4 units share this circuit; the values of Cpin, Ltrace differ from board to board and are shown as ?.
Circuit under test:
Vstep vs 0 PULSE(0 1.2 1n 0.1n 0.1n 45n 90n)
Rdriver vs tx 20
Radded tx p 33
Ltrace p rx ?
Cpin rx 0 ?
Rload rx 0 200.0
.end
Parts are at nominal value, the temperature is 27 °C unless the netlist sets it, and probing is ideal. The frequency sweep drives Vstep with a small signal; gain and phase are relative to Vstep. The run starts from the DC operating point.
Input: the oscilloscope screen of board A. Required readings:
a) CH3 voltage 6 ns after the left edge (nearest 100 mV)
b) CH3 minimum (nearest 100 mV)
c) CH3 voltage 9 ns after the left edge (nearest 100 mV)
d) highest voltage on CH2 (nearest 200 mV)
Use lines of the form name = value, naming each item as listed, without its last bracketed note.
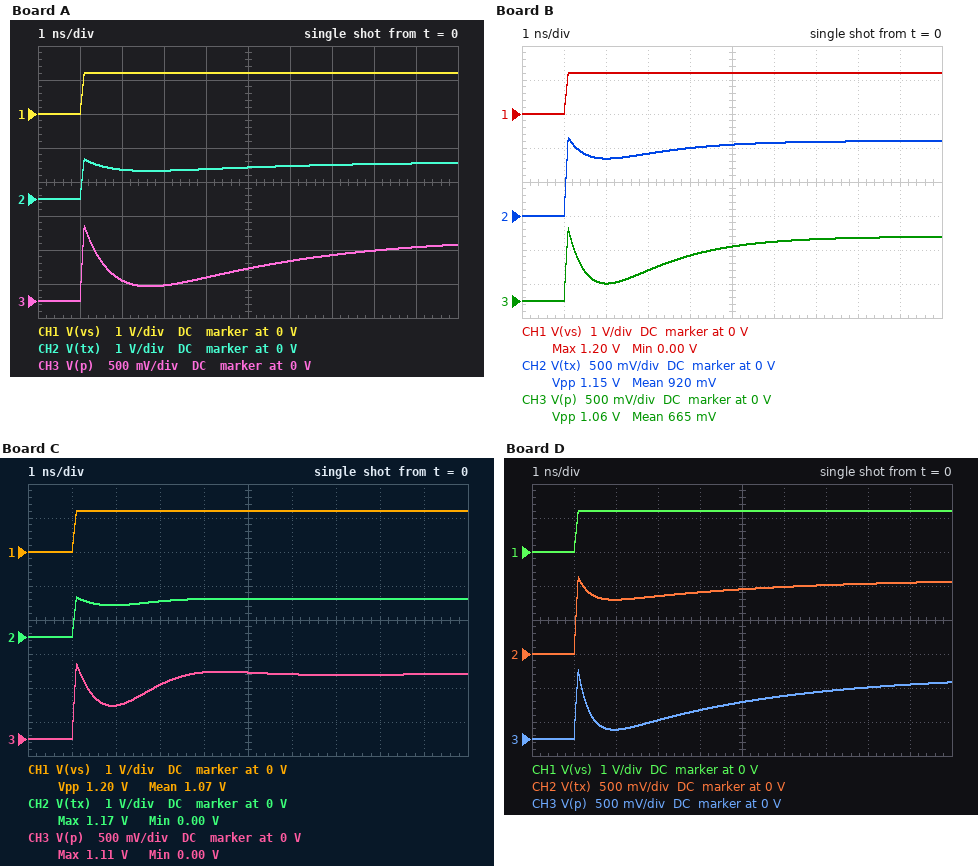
CH3 voltage 6 ns after the left edge = 600 mV
CH3 minimum = 0 V
CH3 voltage 9 ns after the left edge = 800 mV
highest voltage on CH2 = 1.2 V
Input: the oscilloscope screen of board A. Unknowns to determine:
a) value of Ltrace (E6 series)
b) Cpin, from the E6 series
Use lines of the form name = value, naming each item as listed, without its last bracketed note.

value of Ltrace = 33 nH
Cpin, from the E6 series = 100 pF
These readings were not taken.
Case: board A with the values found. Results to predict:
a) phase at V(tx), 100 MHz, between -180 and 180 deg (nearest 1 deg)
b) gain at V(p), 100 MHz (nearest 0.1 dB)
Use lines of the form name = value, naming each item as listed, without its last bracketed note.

phase at V(tx), 100 MHz, between -180 and 180 deg = 3 deg
gain at V(p), 100 MHz = -20.6 dB
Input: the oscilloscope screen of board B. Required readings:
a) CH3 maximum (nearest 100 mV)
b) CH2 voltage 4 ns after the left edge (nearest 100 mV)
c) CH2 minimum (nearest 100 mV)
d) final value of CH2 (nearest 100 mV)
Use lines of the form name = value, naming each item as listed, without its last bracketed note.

CH3 maximum = 1.1 V
CH2 voltage 4 ns after the left edge = 1.0 V
CH2 minimum = 0 V
final value of CH2 = 1.1 V
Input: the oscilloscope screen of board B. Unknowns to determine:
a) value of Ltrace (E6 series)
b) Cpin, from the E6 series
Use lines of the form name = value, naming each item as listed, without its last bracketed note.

value of Ltrace = 22 nH
Cpin, from the E6 series = 47 pF
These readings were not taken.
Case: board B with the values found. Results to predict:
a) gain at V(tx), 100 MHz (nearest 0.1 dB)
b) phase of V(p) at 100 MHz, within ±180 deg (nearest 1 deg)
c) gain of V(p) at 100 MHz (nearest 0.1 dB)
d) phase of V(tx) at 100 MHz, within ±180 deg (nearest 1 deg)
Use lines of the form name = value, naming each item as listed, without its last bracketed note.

gain at V(tx), 100 MHz = -3.1 dB
phase of V(p) at 100 MHz, within ±180 deg = -56 deg
gain of V(p) at 100 MHz = -9.8 dB
phase of V(tx) at 100 MHz, within ±180 deg = -8 deg
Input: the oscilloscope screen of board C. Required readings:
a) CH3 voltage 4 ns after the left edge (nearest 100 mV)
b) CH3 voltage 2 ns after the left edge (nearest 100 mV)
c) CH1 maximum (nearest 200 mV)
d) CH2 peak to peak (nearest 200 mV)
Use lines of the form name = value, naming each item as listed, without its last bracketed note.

CH3 voltage 4 ns after the left edge = 1.0 V
CH3 voltage 2 ns after the left edge = 500 mV
CH1 maximum = 1.2 V
CH2 peak to peak = 1.2 V
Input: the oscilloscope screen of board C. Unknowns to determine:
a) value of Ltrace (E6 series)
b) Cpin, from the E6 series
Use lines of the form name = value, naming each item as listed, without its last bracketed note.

value of Ltrace = 33 nH
Cpin, from the E6 series = 15 pF
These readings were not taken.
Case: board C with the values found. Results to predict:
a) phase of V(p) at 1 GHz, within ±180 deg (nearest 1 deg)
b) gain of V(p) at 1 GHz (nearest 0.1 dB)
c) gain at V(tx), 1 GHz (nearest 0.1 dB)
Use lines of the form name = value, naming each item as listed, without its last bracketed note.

phase of V(p) at 1 GHz, within ±180 deg = 15 deg
gain of V(p) at 1 GHz = -0.3 dB
gain at V(tx), 1 GHz = -0.2 dB
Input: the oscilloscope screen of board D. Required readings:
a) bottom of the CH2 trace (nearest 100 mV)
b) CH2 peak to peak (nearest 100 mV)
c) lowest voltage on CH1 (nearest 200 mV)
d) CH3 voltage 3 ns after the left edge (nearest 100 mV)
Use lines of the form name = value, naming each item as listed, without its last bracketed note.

bottom of the CH2 trace = 0 V
CH2 peak to peak = 1.1 V
lowest voltage on CH1 = 0 V
CH3 voltage 3 ns after the left edge = 300 mV
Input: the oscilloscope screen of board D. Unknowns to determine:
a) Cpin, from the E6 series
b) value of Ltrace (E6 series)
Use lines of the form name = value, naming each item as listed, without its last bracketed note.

Cpin, from the E6 series = 100 pF
value of Ltrace = 15 nH
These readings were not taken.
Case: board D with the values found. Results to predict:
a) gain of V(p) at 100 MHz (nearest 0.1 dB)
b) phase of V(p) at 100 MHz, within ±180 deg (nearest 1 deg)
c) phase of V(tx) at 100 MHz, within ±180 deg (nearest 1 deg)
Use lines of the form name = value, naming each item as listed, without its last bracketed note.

gain of V(p) at 100 MHz = -18.5 dB
phase of V(p) at 100 MHz, within ±180 deg = -72 deg
phase of V(tx) at 100 MHz, within ±180 deg = -4 deg
